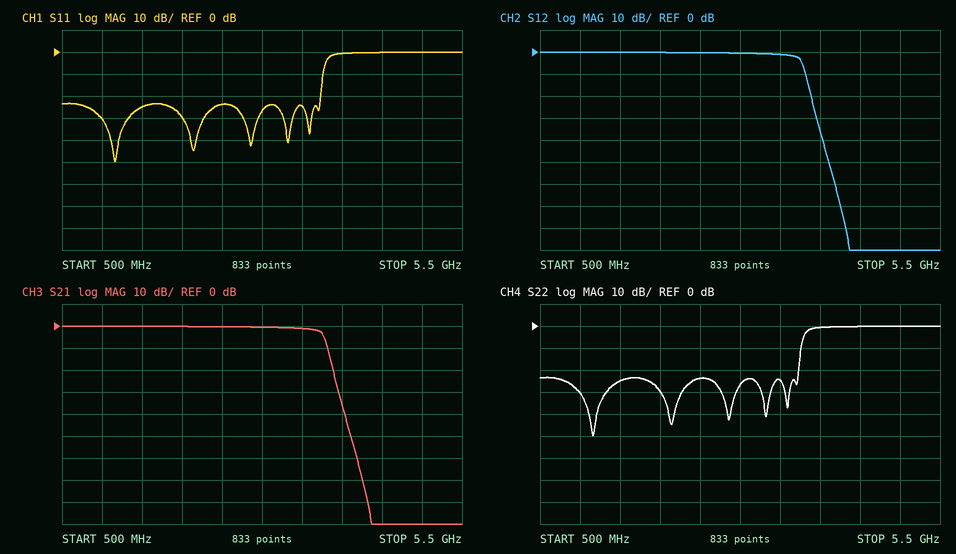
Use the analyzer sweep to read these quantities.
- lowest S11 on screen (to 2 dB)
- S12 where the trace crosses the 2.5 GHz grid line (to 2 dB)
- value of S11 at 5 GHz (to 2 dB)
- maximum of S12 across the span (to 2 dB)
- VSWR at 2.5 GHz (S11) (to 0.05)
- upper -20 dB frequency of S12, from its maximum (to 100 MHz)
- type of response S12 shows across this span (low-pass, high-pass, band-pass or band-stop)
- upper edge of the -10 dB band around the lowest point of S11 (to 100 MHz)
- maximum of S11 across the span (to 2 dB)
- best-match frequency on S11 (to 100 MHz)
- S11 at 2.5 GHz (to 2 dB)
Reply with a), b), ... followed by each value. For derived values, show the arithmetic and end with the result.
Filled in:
a) -50 dB
b) 0 dB
c) 0 dB
d) 0 dB
e) |Γ| = 10^(-24/20) = 0.0631; VSWR = (1 + 0.0631)/(1 − 0.0631) ≈ 1.13, so 1.15 to the nearest 0.05
f) 3.9 GHz
g) low-pass
h) 3.8 GHz
i) 0 dB
j) 1.2 GHz
k) -24 dB
